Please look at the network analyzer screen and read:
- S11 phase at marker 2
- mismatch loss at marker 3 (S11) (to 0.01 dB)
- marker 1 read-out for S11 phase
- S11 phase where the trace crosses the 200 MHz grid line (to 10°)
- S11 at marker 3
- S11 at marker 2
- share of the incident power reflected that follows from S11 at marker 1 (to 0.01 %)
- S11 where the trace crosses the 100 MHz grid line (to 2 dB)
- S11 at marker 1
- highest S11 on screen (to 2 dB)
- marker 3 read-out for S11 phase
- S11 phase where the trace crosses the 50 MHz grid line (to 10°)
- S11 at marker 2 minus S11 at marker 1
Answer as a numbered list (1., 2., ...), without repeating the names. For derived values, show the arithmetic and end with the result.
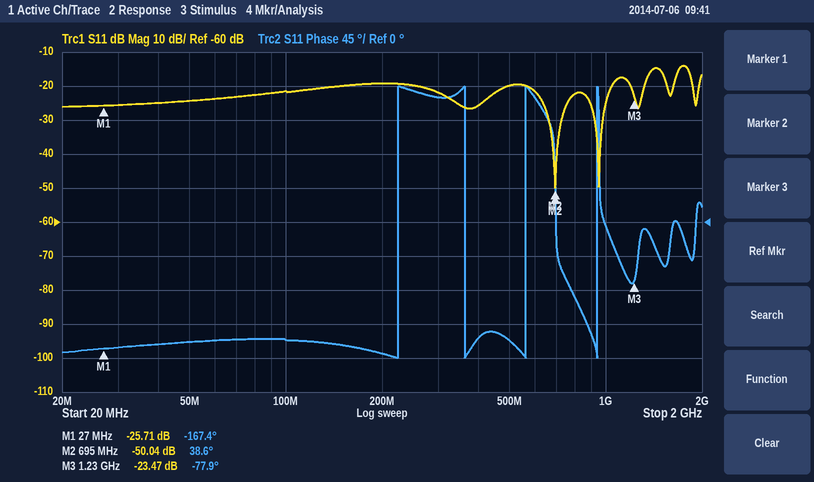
1. 38.6°
2. −10 log10(1 − 10^(-23.47/10)) ≈ 0.02 dB
3. -167.4°
4. -170°
5. -23.47 dB
6. -50.04 dB
7. 10^(-25.71/10) ≈ 0.27 %
8. -22 dB
9. -25.71 dB
10. -14 dB
11. -77.9°
12. -160°
13. -50.04 − (-25.71) = -24.33 dB
